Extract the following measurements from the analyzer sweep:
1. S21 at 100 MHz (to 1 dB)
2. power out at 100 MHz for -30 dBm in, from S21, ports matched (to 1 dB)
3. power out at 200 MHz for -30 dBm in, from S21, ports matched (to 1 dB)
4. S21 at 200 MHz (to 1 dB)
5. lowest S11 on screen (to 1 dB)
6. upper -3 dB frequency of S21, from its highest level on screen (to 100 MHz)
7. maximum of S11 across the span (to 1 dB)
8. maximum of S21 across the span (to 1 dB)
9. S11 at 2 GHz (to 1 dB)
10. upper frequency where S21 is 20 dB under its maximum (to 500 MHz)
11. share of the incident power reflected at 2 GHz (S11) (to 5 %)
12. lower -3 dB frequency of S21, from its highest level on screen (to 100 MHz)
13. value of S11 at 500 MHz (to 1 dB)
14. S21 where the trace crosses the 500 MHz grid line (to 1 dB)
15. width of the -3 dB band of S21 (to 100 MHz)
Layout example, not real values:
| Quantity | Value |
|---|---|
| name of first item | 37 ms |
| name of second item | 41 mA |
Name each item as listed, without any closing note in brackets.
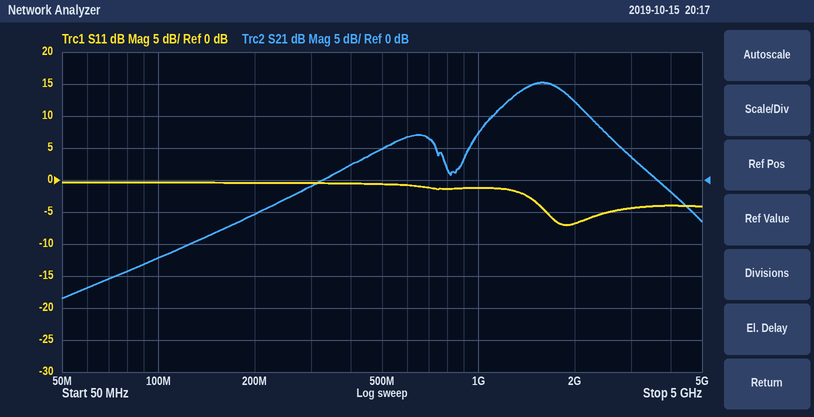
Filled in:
| Quantity | Value |
|---|---|
| S21 at 100 MHz | -12 dB |
| power out at 100 MHz for -30 dBm in, from S21, ports matched | -42 dBm |
| power out at 200 MHz for -30 dBm in, from S21, ports matched | -35 dBm |
| S21 at 200 MHz | -5 dB |
| lowest S11 on screen | -7 dB |
| upper -3 dB frequency of S21, from its highest level on screen | 2.0 GHz |
| maximum of S11 across the span | 0 dB |
| maximum of S21 across the span | 15 dB |
| S11 at 2 GHz | -7 dB |
| upper frequency where S21 is 20 dB under its maximum | 4.5 GHz |
| share of the incident power reflected at 2 GHz (S11) | 20 % |
| lower -3 dB frequency of S21, from its highest level on screen | 1.2 GHz |
| value of S11 at 500 MHz | -1 dB |
| S21 where the trace crosses the 500 MHz grid line | 5 dB |
| width of the -3 dB band of S21 | 800 MHz |
